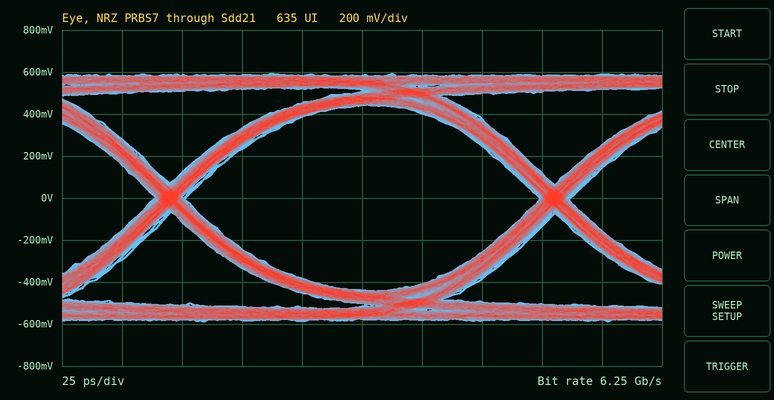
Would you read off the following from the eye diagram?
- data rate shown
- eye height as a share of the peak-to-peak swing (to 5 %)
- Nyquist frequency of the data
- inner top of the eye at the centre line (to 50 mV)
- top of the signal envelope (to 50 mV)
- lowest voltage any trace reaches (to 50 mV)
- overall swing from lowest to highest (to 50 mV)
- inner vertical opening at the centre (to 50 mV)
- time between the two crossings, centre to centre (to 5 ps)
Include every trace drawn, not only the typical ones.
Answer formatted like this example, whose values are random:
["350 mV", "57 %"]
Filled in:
["6.25 Gb/s", "75 %", "3.125 GHz", "450 mV", "600 mV", "-600 mV", "1.20 V", "900 mV", "160 ps"]
